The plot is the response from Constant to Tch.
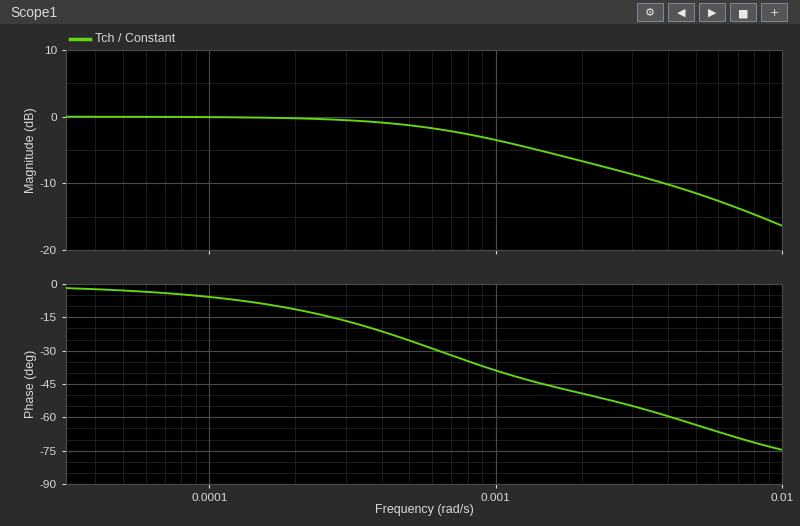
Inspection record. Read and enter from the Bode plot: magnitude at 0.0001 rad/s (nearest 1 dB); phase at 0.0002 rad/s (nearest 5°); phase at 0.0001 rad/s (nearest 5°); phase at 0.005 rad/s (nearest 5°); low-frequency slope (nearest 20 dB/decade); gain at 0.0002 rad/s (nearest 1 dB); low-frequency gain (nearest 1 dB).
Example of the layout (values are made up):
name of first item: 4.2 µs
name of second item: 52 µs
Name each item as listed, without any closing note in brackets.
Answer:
magnitude at 0.0001 rad/s: 0 dB
phase at 0.0002 rad/s: -10°
phase at 0.0001 rad/s: -5°
phase at 0.005 rad/s: -65°
low-frequency slope: 0 dB/decade
gain at 0.0002 rad/s: 0 dB
low-frequency gain: 0 dB
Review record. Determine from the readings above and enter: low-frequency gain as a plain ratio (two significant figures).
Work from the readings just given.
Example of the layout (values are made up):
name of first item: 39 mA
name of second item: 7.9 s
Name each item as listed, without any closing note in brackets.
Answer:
low-frequency gain as a plain ratio: 1.0
